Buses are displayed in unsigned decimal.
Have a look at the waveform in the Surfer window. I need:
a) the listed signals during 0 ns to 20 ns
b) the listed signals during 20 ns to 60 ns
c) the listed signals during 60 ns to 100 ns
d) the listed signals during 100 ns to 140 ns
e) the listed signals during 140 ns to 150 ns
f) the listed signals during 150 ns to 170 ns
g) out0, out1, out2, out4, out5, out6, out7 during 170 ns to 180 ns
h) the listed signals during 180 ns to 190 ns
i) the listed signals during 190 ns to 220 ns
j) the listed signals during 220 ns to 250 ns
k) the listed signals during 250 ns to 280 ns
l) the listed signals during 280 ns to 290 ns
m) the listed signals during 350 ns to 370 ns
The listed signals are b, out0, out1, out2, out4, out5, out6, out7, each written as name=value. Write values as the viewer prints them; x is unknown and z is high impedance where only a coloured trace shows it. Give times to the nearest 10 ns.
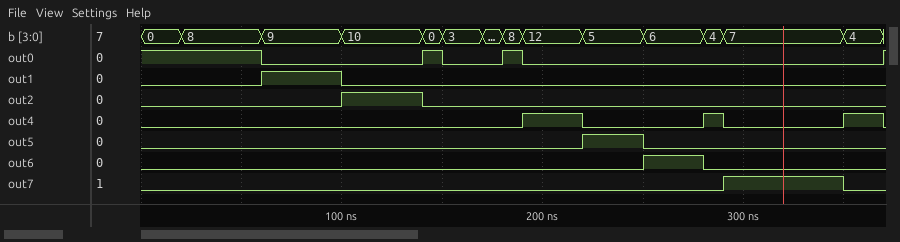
b=0, out0=1, out1=0, out2=0, out4=0, out5=0, out6=0, out7=0
b=8, out0=1, out1=0, out2=0, out4=0, out5=0, out6=0, out7=0
b=9, out0=0, out1=1, out2=0, out4=0, out5=0, out6=0, out7=0
b=10, out0=0, out1=0, out2=1, out4=0, out5=0, out6=0, out7=0
b=0, out0=1, out1=0, out2=0, out4=0, out5=0, out6=0, out7=0
b=3, out0=0, out1=0, out2=0, out4=0, out5=0, out6=0, out7=0
out0=0, out1=0, out2=0, out4=0, out5=0, out6=0, out7=0
b=8, out0=1, out1=0, out2=0, out4=0, out5=0, out6=0, out7=0
b=12, out0=0, out1=0, out2=0, out4=1, out5=0, out6=0, out7=0
b=5, out0=0, out1=0, out2=0, out4=0, out5=1, out6=0, out7=0
b=6, out0=0, out1=0, out2=0, out4=0, out5=0, out6=1, out7=0
b=4, out0=0, out1=0, out2=0, out4=1, out5=0, out6=0, out7=0
b=4, out0=0, out1=0, out2=0, out4=1, out5=0, out6=0, out7=0
